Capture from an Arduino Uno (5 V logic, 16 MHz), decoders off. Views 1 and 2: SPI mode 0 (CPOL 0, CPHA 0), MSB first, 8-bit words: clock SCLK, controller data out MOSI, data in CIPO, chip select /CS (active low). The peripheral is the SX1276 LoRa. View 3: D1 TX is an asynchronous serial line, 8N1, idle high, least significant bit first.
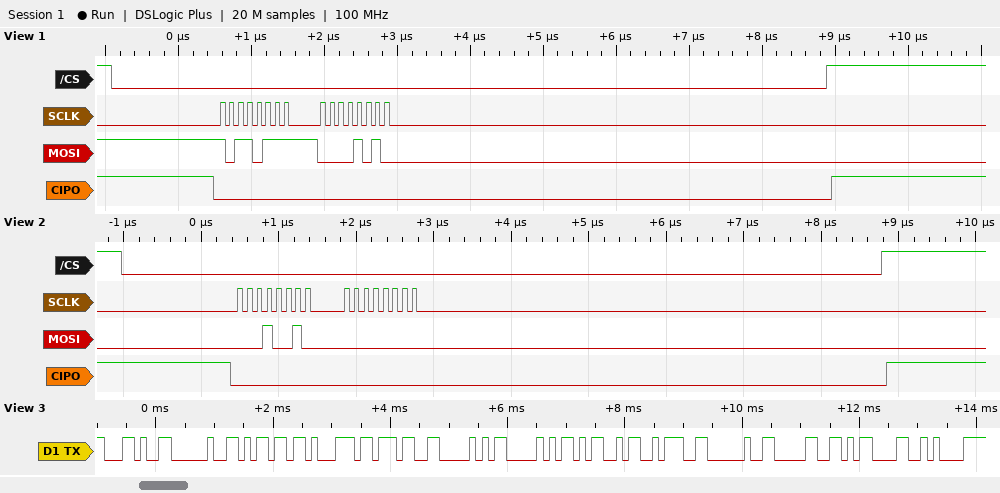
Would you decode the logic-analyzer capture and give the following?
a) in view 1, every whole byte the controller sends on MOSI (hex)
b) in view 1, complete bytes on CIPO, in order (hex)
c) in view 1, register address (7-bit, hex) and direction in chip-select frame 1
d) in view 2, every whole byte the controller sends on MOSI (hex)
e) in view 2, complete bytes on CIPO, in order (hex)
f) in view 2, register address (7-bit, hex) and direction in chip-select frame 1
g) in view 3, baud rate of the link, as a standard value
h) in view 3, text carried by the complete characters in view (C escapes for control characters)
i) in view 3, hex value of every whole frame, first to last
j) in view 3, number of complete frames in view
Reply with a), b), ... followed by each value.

a) B7 0A
b) 00 00
c) 0x37 write
d) 0x12 0x00
e) 0x00 0x00
f) 0x12 read
g) 9600 baud
h) ", mq7PPM: 0\r\n"
i) 0x2C 0x20 0x6D 0x71 0x37 0x50 0x50 0x4D 0x3A 0x20 0x30 0x0D 0x0A
j) 13
